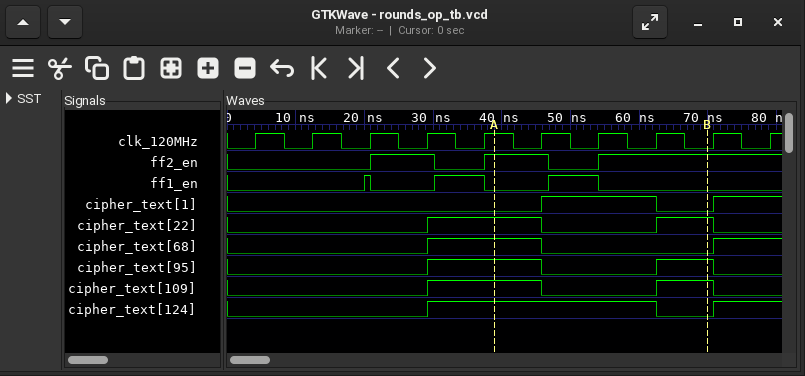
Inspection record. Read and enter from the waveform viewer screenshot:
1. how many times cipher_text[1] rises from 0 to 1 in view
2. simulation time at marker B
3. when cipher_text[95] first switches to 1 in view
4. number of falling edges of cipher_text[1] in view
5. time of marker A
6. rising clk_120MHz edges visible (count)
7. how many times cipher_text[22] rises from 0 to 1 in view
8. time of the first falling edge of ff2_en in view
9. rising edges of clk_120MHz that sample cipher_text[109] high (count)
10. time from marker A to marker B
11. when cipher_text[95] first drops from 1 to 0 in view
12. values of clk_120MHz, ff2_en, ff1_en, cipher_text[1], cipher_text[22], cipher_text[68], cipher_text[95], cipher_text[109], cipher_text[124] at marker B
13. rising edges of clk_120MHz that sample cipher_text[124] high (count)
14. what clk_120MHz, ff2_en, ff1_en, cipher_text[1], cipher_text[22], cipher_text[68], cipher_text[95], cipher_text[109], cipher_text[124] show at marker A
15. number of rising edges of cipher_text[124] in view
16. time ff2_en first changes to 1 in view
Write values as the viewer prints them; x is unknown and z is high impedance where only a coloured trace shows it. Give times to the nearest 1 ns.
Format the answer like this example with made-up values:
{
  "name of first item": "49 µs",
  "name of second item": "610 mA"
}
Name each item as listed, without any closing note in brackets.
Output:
{
  "how many times cipher_text[1] rises from 0 to 1 in view": "2",
  "simulation time at marker B": "70 ns",
  "when cipher_text[95] first switches to 1 in view": "29 ns",
  "number of falling edges of cipher_text[1] in view": "1",
  "time of marker A": "39 ns",
  "rising clk_120MHz edges visible": "10",
  "how many times cipher_text[22] rises from 0 to 1 in view": "2",
  "time of the first falling edge of ff2_en in view": "30 ns",
  "rising edges of clk_120MHz that sample cipher_text[109] high": "3",
  "time from marker A to marker B": "31 ns",
  "when cipher_text[95] first drops from 1 to 0 in view": "46 ns",
  "values of clk_120MHz, ff2_en, ff1_en, cipher_text[1], cipher_text[22], cipher_text[68], cipher_text[95], cipher_text[109], cipher_text[124] at marker B": "clk_120MHz=0, ff2_en=1, ff1_en=0, cipher_text[1]=0, cipher_text[22]=1, cipher_text[68]=0, cipher_text[95]=1, cipher_text[109]=1, cipher_text[124]=0",
  "rising edges of clk_120MHz that sample cipher_text[124] high": "5",
  "what clk_120MHz, ff2_en, ff1_en, cipher_text[1], cipher_text[22], cipher_text[68], cipher_text[95], cipher_text[109], cipher_text[124] show at marker A": "clk_120MHz=1, ff2_en=1, ff1_en=0, cipher_text[1]=0, cipher_text[22]=1, cipher_text[68]=1, cipher_text[95]=1, cipher_text[109]=1, cipher_text[124]=1",
  "number of rising edges of cipher_text[124] in view": "2",
  "time ff2_en first changes to 1 in view": "21 ns"
}
